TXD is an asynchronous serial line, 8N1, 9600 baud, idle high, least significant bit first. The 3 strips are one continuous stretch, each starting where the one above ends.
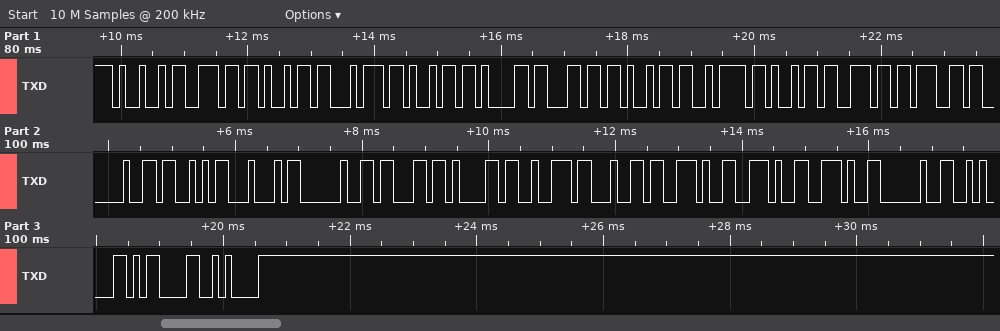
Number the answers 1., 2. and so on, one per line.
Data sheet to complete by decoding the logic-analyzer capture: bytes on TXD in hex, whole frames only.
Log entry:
1. 49 6E 69 74 69 61 6C 69 7A 69 6E 67 20 53 44 20 63 61 72 64 2E 2E 2E 20 0A 0D 0A
